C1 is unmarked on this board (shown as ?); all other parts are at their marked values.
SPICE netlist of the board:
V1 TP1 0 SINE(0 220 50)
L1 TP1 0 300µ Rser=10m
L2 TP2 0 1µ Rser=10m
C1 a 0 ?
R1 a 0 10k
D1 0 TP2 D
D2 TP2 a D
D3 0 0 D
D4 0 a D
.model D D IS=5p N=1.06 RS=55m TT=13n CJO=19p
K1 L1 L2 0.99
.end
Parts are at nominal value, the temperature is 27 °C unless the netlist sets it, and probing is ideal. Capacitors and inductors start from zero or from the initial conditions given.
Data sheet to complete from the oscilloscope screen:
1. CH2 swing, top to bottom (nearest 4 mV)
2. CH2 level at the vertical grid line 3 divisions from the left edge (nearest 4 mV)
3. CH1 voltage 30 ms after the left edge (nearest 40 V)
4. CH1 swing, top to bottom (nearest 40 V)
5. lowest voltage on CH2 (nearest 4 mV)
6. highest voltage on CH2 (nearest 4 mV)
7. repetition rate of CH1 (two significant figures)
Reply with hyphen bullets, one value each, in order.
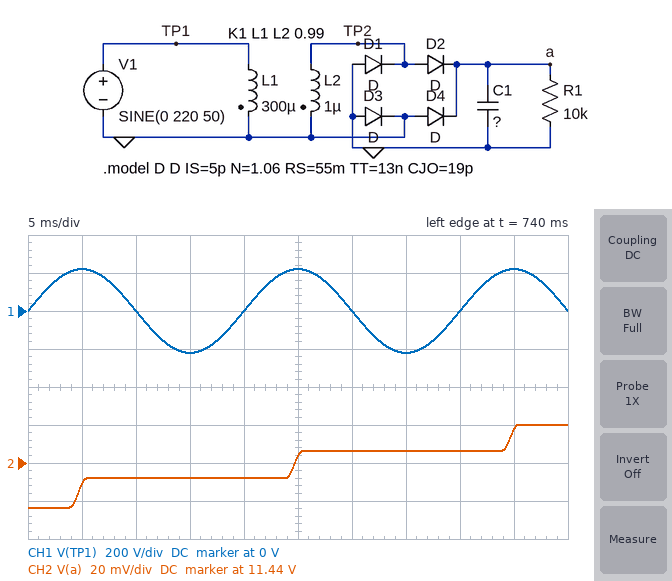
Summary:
- 44 mV
- 11.432 V
- 0 V
- 440 V
- 11.416 V
- 11.460 V
- 50 Hz
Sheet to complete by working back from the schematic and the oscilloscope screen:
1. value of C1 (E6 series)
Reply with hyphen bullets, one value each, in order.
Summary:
- 330 mF
